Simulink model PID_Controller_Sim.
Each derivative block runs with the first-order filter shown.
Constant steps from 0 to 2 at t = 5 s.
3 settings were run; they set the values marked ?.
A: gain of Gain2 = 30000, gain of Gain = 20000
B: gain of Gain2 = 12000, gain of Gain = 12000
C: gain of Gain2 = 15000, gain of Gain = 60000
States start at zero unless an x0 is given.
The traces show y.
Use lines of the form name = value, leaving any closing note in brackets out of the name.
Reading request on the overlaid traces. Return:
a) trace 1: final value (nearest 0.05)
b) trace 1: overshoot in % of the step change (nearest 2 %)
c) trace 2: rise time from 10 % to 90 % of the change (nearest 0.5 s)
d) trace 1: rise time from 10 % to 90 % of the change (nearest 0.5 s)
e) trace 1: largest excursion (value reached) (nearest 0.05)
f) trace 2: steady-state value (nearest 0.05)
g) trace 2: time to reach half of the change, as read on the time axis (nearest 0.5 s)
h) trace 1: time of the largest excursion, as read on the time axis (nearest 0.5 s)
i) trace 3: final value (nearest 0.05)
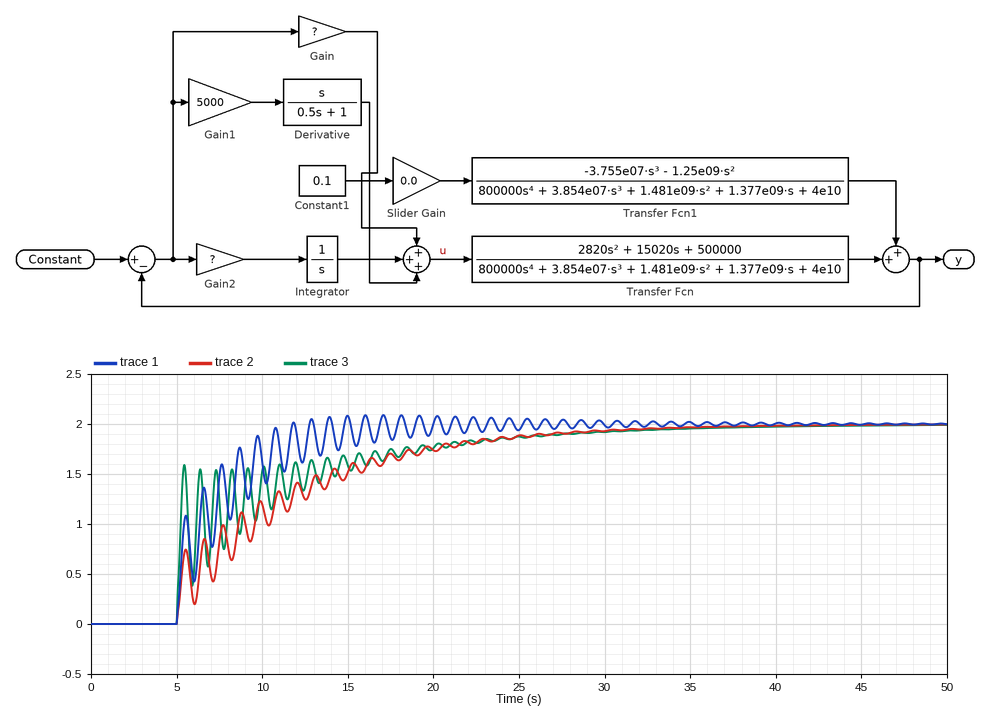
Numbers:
trace 1: final value = 2.00
trace 1: overshoot in % of the step change = 4 %
trace 2: rise time from 10 % to 90 % of the change = 15.5 s
trace 1: rise time from 10 % to 90 % of the change = 4.5 s
trace 1: largest excursion (value reached) = 2.10
trace 2: steady-state value = 2.00
trace 2: time to reach half of the change, as read on the time axis = 8.5 s
trace 1: time of the largest excursion, as read on the time axis = 17.0 s
trace 3: final value = 2.00
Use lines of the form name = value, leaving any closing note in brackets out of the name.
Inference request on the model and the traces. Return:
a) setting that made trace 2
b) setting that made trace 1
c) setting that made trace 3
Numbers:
setting that made trace 2 = B
setting that made trace 1 = A
setting that made trace 3 = C
